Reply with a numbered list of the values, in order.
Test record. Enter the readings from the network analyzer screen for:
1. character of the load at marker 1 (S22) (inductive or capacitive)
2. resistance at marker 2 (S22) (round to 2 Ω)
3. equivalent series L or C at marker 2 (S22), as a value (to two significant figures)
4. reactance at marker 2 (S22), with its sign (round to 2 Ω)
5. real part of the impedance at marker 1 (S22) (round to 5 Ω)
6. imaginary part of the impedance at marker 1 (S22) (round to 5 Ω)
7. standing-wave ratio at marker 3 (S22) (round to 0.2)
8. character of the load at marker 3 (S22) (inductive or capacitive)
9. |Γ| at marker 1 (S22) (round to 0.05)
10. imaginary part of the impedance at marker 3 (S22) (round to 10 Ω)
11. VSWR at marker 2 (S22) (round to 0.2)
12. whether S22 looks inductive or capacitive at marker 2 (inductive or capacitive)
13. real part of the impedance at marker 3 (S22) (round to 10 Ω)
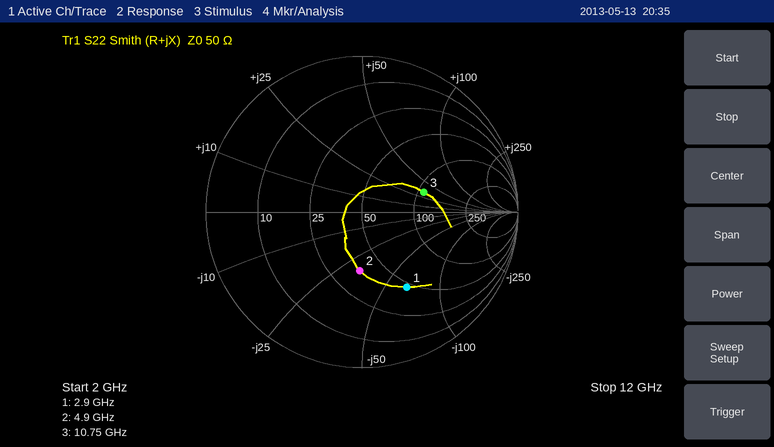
1. capacitive
2. 36 Ω
3. 1.0 pF
4. -32 Ω
5. 45 Ω
6. -65 Ω
7. 2.4
8. inductive
9. 0.55
10. +30 Ω
11. 2.2
12. capacitive
13. 110 Ω
